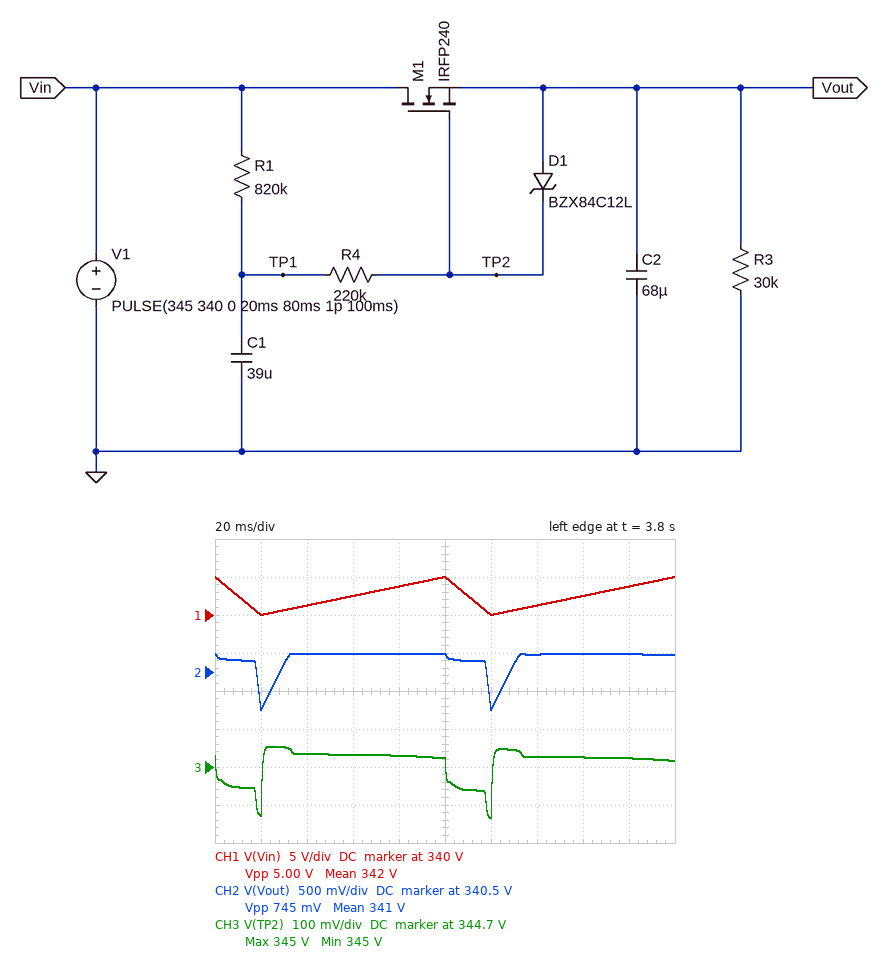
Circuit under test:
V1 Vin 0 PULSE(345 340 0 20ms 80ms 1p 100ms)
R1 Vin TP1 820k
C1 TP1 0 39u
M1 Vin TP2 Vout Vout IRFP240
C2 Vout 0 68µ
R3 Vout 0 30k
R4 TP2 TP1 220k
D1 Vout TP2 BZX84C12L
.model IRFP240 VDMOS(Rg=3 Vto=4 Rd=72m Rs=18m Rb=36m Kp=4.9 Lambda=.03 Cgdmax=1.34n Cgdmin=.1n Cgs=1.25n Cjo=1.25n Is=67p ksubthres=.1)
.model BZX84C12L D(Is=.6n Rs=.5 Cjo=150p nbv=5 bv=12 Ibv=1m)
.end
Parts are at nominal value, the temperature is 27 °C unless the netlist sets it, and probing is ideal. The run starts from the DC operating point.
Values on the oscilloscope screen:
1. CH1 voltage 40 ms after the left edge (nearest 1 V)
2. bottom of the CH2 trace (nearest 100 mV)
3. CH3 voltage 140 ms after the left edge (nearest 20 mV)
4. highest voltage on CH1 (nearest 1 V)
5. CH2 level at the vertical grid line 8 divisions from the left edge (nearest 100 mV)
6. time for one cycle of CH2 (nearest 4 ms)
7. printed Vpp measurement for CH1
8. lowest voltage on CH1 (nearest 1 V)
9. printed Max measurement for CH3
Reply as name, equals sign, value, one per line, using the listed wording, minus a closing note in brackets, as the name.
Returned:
CH1 voltage 40 ms after the left edge = 341 V
bottom of the CH2 trace = 340.0 V
CH3 voltage 140 ms after the left edge = 344.72 V
highest voltage on CH1 = 345 V
CH2 level at the vertical grid line 8 divisions from the left edge = 340.7 V
time for one cycle of CH2 = 100 ms
printed Vpp measurement for CH1 = 5.00 V
lowest voltage on CH1 = 340 V
printed Max measurement for CH3 = 345 V
